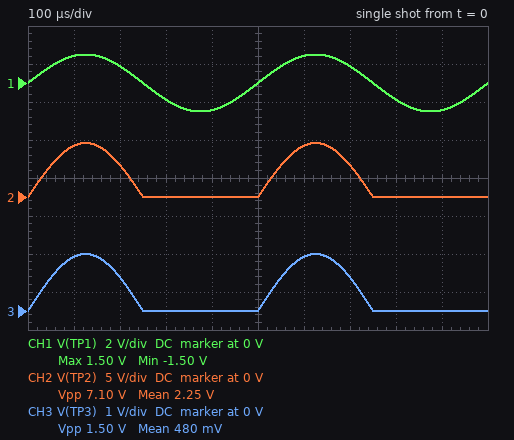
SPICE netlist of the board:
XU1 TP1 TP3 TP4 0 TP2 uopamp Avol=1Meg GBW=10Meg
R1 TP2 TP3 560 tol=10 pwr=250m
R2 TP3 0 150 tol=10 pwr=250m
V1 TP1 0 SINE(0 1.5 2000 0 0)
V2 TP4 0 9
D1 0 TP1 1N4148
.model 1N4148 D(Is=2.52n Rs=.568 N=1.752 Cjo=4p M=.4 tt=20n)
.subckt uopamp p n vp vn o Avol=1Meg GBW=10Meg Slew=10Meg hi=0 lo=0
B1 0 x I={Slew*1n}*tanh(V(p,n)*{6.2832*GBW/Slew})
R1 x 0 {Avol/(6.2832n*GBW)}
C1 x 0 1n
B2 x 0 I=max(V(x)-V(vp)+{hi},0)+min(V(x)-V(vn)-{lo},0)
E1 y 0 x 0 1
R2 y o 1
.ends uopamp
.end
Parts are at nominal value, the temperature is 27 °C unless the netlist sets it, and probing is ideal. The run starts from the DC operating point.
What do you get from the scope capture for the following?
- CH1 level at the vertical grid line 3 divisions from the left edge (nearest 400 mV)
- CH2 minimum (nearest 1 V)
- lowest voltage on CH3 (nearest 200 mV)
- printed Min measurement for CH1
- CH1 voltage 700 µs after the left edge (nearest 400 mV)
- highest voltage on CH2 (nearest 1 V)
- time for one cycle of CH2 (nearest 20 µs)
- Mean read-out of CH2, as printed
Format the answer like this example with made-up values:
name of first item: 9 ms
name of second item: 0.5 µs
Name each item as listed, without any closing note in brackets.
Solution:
CH1 level at the vertical grid line 3 divisions from the left edge: -800 mV
CH2 minimum: 0 V
lowest voltage on CH3: 0 V
printed Min measurement for CH1: -1.50 V
CH1 voltage 700 µs after the left edge: 800 mV
highest voltage on CH2: 7 V
time for one cycle of CH2: 500 µs
Mean read-out of CH2, as printed: 2.25 V
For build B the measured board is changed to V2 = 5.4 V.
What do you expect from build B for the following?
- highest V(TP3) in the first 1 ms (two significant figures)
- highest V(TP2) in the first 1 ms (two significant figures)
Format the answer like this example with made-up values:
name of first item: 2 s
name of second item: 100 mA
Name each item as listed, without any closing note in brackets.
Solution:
highest V(TP3) in the first 1 ms: 1.1 V
highest V(TP2) in the first 1 ms: 5.4 V
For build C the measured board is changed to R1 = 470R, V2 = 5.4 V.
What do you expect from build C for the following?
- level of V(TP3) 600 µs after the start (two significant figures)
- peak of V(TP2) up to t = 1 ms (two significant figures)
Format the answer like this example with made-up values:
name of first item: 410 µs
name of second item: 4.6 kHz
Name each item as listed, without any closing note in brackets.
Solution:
level of V(TP3) 600 µs after the start: 1.3 V
peak of V(TP2) up to t = 1 ms: 5.4 V
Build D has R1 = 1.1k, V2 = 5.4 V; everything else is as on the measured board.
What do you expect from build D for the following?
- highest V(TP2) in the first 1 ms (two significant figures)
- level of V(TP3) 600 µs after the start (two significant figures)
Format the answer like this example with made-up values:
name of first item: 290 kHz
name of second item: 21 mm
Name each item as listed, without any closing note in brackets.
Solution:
highest V(TP2) in the first 1 ms: 5.4 V
level of V(TP3) 600 µs after the start: 650 mV
